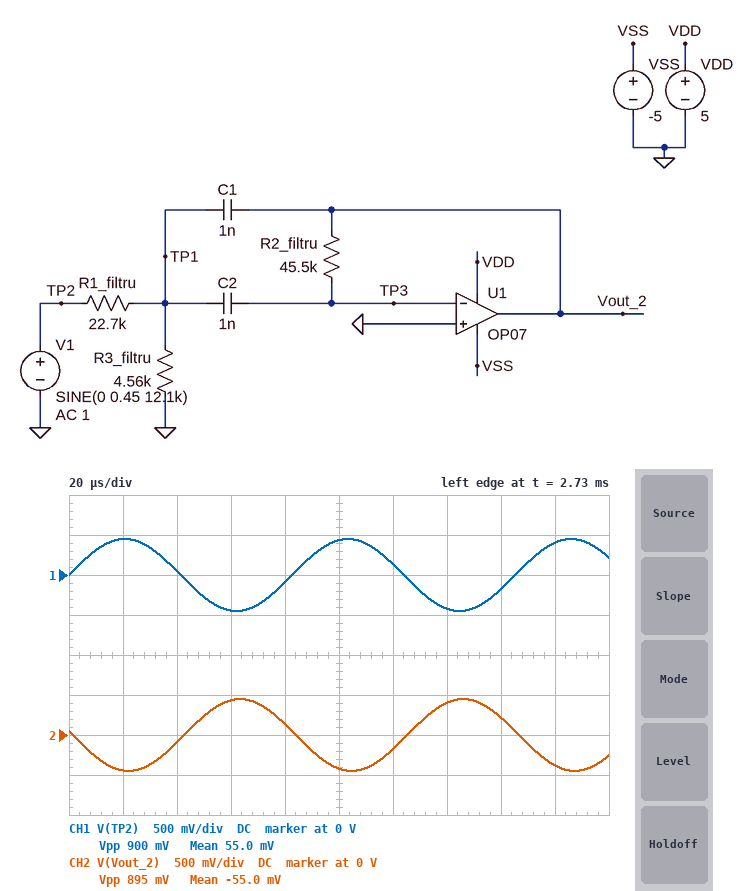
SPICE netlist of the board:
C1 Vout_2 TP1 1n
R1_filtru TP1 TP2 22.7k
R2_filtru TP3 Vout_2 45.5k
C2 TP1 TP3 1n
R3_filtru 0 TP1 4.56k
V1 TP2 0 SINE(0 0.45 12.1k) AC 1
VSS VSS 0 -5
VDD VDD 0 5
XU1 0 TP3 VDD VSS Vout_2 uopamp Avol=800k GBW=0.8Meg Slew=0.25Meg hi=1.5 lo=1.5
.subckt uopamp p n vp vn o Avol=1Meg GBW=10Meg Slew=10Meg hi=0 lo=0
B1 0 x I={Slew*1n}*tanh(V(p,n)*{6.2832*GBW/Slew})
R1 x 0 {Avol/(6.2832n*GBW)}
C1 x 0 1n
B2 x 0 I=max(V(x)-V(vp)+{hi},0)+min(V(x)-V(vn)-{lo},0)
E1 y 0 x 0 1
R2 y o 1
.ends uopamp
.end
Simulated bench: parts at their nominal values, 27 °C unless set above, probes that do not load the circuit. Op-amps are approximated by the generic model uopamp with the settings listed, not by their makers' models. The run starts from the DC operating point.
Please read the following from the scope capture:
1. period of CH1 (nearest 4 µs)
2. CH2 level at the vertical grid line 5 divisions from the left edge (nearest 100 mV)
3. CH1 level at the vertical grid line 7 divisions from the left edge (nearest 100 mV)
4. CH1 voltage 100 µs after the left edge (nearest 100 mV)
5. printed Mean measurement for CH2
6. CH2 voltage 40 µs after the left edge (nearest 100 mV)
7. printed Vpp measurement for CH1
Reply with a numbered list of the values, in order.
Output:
1. 84 µs
2. -400 mV
3. -400 mV
4. 400 mV
5. -55.0 mV
6. -100 mV
7. 900 mV
